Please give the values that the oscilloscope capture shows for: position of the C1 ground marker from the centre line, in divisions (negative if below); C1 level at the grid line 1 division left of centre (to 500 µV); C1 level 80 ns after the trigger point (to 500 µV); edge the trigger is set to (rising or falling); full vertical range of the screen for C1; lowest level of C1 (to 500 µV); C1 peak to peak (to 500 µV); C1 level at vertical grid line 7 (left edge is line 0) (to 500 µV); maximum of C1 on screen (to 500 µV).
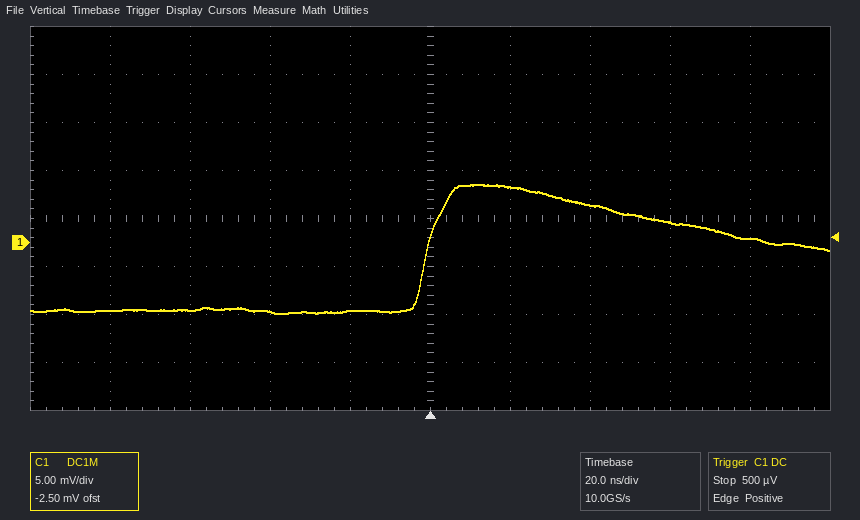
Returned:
-0.5 div
-7.0 mV
500 µV
rising
40 mV
-7.5 mV
13.5 mV
4.0 mV
6.0 mV
